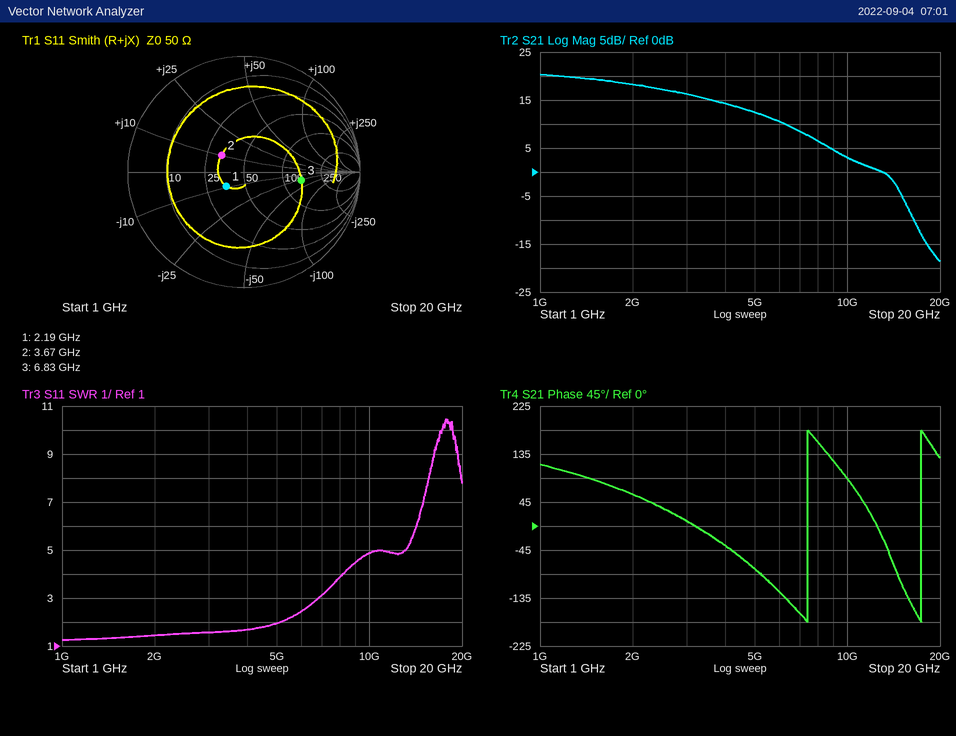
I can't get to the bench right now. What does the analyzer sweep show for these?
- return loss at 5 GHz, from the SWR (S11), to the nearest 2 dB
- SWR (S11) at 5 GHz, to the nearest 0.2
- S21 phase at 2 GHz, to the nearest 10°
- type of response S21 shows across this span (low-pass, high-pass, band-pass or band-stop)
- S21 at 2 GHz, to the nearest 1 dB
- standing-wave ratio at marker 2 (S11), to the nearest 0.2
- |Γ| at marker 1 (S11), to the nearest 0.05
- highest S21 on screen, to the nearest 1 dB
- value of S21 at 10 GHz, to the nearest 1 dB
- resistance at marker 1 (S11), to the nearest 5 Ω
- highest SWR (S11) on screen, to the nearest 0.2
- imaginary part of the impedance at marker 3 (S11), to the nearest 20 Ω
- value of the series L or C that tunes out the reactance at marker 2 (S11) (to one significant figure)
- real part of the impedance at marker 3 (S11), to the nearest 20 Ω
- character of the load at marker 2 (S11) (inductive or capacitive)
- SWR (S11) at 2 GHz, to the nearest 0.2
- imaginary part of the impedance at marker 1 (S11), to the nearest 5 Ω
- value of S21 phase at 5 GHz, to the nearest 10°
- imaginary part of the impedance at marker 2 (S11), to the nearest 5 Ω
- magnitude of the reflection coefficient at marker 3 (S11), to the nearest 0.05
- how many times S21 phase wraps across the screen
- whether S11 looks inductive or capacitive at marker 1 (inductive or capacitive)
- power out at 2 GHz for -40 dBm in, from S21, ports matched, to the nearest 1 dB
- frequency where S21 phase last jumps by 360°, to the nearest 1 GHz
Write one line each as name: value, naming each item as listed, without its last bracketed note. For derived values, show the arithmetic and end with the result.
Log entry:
return loss at 5 GHz, from the SWR (S11), to the nearest 2 dB: −20 log10((2 − 1)/(2 + 1)) ≈ 10 dB
SWR (S11) at 5 GHz, to the nearest 0.2: 2.0
S21 phase at 2 GHz, to the nearest 10°: 60°
type of response S21 shows across this span: low-pass
S21 at 2 GHz, to the nearest 1 dB: 18 dB
standing-wave ratio at marker 2 (S11), to the nearest 0.2: 1.6
|Γ| at marker 1 (S11), to the nearest 0.05: 0.20
highest S21 on screen, to the nearest 1 dB: 20 dB
value of S21 at 10 GHz, to the nearest 1 dB: 3 dB
resistance at marker 1 (S11), to the nearest 5 Ω: 35 Ω
highest SWR (S11) on screen, to the nearest 0.2: 10.4
imaginary part of the impedance at marker 3 (S11), to the nearest 20 Ω: -20 Ω
value of the series L or C that tunes out the reactance at marker 2 (S11): C = 1/(2π × 3.67 GHz × 10 Ω) ≈ 4 pF
real part of the impedance at marker 3 (S11), to the nearest 20 Ω: 140 Ω
character of the load at marker 2 (S11): inductive
SWR (S11) at 2 GHz, to the nearest 0.2: 1.4
imaginary part of the impedance at marker 1 (S11), to the nearest 5 Ω: -10 Ω
value of S21 phase at 5 GHz, to the nearest 10°: -80°
imaginary part of the impedance at marker 2 (S11), to the nearest 5 Ω: +10 Ω
magnitude of the reflection coefficient at marker 3 (S11), to the nearest 0.05: 0.50
how many times S21 phase wraps across the screen: 2
whether S11 looks inductive or capacitive at marker 1: capacitive
power out at 2 GHz for -40 dBm in, from S21, ports matched, to the nearest 1 dB: -40 dBm + (18 dB) = -22 dBm
frequency where S21 phase last jumps by 360°, to the nearest 1 GHz: 17 GHz
